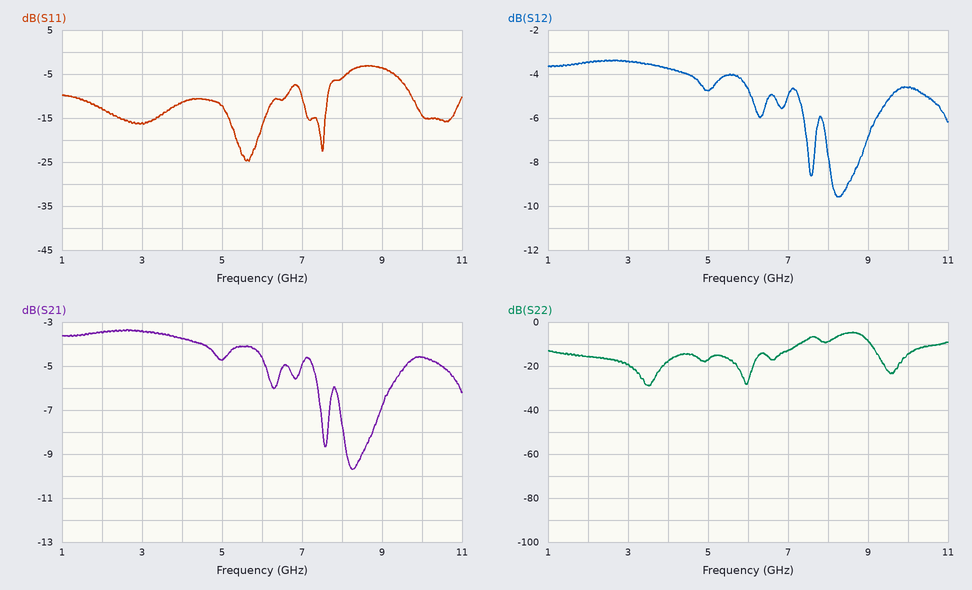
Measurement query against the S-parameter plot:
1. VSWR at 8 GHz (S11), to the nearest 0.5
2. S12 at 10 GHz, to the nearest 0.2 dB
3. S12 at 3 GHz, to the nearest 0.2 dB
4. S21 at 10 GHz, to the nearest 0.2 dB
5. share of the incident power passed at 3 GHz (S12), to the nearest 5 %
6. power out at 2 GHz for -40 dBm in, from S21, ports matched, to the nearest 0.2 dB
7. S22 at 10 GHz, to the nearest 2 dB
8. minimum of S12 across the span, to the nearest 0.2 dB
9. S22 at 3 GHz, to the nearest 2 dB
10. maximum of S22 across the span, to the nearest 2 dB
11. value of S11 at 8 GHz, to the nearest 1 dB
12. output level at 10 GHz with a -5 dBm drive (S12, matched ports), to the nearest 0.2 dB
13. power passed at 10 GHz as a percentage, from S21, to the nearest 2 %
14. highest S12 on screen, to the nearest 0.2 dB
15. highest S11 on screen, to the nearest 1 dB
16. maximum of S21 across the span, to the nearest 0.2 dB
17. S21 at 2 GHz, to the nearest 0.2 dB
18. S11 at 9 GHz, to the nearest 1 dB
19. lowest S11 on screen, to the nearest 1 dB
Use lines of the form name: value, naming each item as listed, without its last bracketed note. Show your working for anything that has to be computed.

VSWR at 8 GHz (S11), to the nearest 0.5: |Γ| = 10^(-6/20) = 0.5012; VSWR = (1 + 0.5012)/(1 − 0.5012) ≈ 3.0
S12 at 10 GHz, to the nearest 0.2 dB: -4.6 dB
S12 at 3 GHz, to the nearest 0.2 dB: -3.4 dB
S21 at 10 GHz, to the nearest 0.2 dB: -4.6 dB
share of the incident power passed at 3 GHz (S12), to the nearest 5 %: 10^(-3.4/10) ≈ 45.7 %, so 45 % to the nearest 5 %
power out at 2 GHz for -40 dBm in, from S21, ports matched, to the nearest 0.2 dB: -40 dBm + (-3.4 dB) = -43.4 dBm
S22 at 10 GHz, to the nearest 2 dB: -14 dB
minimum of S12 across the span, to the nearest 0.2 dB: -9.6 dB
S22 at 3 GHz, to the nearest 2 dB: -20 dB
maximum of S22 across the span, to the nearest 2 dB: -4 dB
value of S11 at 8 GHz, to the nearest 1 dB: -6 dB
output level at 10 GHz with a -5 dBm drive (S12, matched ports), to the nearest 0.2 dB: -5 dBm + (-4.6 dB) = -9.6 dBm
power passed at 10 GHz as a percentage, from S21, to the nearest 2 %: 10^(-4.6/10) ≈ 34.7 %, so 34 % to the nearest 2 %
highest S12 on screen, to the nearest 0.2 dB: -3.4 dB
highest S11 on screen, to the nearest 1 dB: -3 dB
maximum of S21 across the span, to the nearest 0.2 dB: -3.4 dB
S21 at 2 GHz, to the nearest 0.2 dB: -3.4 dB
S11 at 9 GHz, to the nearest 1 dB: -4 dB
lowest S11 on screen, to the nearest 1 dB: -25 dB
